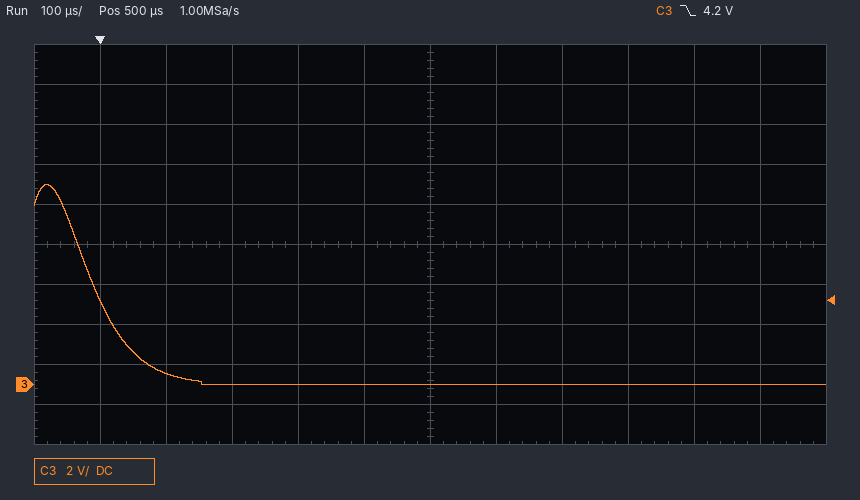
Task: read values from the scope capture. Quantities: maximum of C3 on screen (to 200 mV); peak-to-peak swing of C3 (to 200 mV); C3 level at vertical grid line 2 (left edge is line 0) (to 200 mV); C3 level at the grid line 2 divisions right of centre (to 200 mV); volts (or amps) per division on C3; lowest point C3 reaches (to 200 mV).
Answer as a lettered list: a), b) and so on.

a) 10.0 V
b) 10.0 V
c) 600 mV
d) 0.0 V
e) 2 V
f) 0.0 V
